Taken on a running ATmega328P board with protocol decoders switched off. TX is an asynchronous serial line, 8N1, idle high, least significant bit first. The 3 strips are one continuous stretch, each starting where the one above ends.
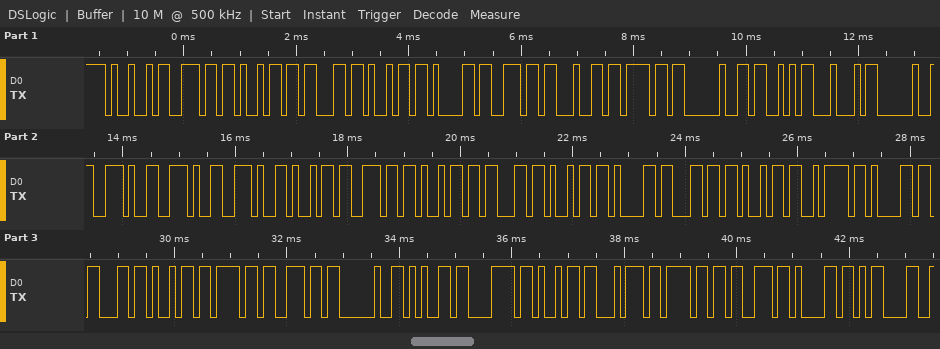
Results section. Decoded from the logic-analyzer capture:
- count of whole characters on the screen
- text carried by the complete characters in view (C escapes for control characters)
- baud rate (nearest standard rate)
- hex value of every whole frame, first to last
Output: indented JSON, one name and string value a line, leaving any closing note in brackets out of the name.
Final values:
{
  "count of whole characters on the screen": "39",
  "text carried by the complete characters in view": "\"Iniciando SD ...inicializacion exitosa\\r\"",
  "baud rate": "9600 baud",
  "hex value of every whole frame, first to last": "49 6E 69 63 69 61 6E 64 6F 20 53 44 20 2E 2E 2E 69 6E 69 63 69 61 6C 69 7A 61 63 69 6F 6E 20 65 78 69 74 6F 73 61 0D"
}
